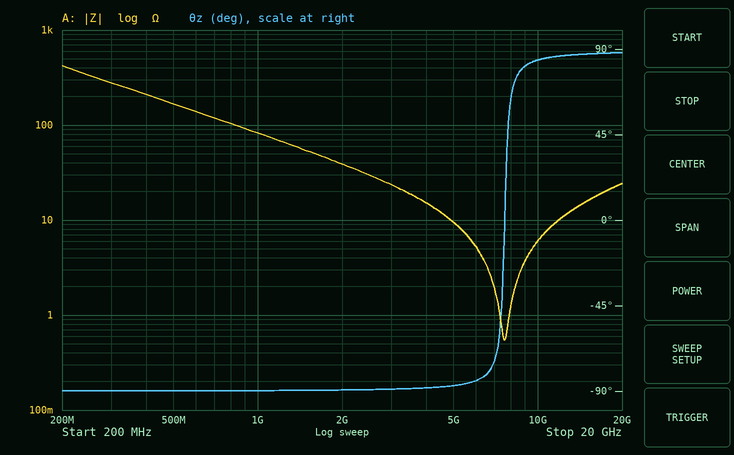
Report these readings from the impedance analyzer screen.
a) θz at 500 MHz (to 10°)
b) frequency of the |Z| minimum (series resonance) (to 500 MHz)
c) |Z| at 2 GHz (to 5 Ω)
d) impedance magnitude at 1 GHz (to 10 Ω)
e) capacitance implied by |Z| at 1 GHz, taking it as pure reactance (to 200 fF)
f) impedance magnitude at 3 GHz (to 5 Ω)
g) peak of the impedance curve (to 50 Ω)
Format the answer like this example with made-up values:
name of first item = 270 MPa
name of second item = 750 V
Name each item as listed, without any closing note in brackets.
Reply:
θz at 500 MHz = -90°
frequency of the |Z| minimum (series resonance) = 7.5 GHz
|Z| at 2 GHz = 40 Ω
impedance magnitude at 1 GHz = 80 Ω
capacitance implied by |Z| at 1 GHz, taking it as pure reactance = 2.0 pF
impedance magnitude at 3 GHz = 25 Ω
peak of the impedance curve = 400 Ω
